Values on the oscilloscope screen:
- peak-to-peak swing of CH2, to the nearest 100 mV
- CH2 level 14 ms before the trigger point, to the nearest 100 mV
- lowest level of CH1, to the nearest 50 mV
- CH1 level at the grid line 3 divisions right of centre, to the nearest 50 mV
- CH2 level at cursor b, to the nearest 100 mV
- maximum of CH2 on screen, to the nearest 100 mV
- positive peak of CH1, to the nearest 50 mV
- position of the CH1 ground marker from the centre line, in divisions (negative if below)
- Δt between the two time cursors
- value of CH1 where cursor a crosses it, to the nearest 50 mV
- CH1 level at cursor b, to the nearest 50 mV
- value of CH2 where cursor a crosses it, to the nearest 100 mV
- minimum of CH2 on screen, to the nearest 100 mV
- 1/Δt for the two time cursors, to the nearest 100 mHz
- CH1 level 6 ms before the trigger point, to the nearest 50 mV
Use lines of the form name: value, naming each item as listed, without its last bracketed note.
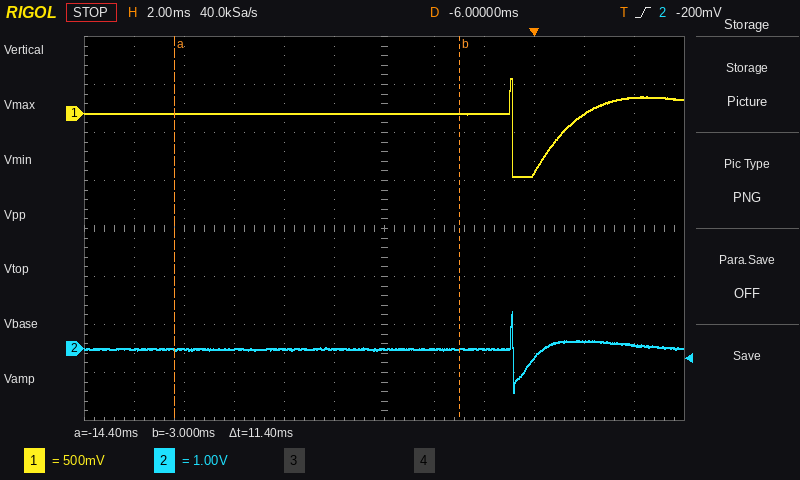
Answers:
peak-to-peak swing of CH2, to the nearest 100 mV: 1.7 V
CH2 level 14 ms before the trigger point, to the nearest 100 mV: 0.0 V
lowest level of CH1, to the nearest 50 mV: -650 mV
CH1 level at the grid line 3 divisions right of centre, to the nearest 50 mV: -600 mV
CH2 level at cursor b, to the nearest 100 mV: 0.0 V
maximum of CH2 on screen, to the nearest 100 mV: 800 mV
positive peak of CH1, to the nearest 50 mV: 350 mV
position of the CH1 ground marker from the centre line, in divisions: +2.4 div
Δt between the two time cursors: 11.4 ms
value of CH1 where cursor a crosses it, to the nearest 50 mV: 0 mV
CH1 level at cursor b, to the nearest 50 mV: 0 mV
value of CH2 where cursor a crosses it, to the nearest 100 mV: 0.0 V
minimum of CH2 on screen, to the nearest 100 mV: -900 mV
1/Δt for the two time cursors, to the nearest 100 mHz: 87.7 Hz
CH1 level 6 ms before the trigger point, to the nearest 50 mV: 0 mV
